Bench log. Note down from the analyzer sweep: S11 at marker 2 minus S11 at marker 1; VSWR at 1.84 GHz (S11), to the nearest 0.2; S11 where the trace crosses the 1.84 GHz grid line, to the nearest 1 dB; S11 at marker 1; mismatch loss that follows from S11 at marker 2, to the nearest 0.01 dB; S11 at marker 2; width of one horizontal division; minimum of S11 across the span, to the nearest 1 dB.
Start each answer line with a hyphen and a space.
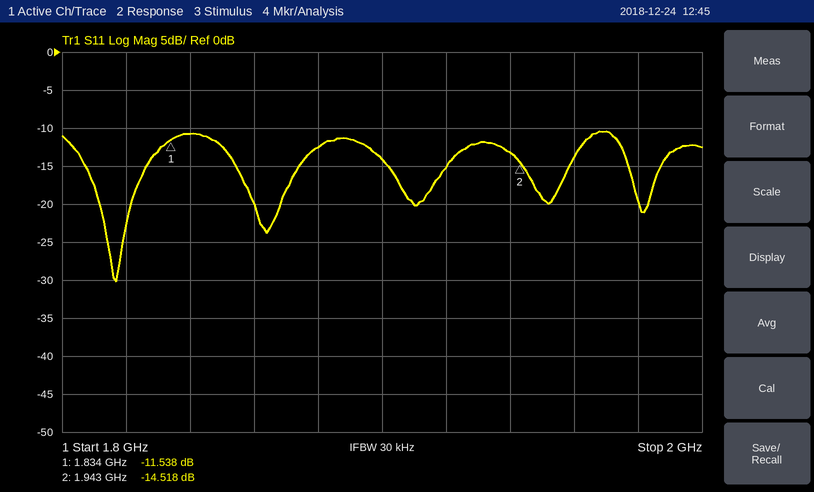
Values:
- -2.980 dB
- 1.8
- -11 dB
- -11.538 dB
- 0.16 dB
- -14.518 dB
- 20 MHz
- -30 dB
